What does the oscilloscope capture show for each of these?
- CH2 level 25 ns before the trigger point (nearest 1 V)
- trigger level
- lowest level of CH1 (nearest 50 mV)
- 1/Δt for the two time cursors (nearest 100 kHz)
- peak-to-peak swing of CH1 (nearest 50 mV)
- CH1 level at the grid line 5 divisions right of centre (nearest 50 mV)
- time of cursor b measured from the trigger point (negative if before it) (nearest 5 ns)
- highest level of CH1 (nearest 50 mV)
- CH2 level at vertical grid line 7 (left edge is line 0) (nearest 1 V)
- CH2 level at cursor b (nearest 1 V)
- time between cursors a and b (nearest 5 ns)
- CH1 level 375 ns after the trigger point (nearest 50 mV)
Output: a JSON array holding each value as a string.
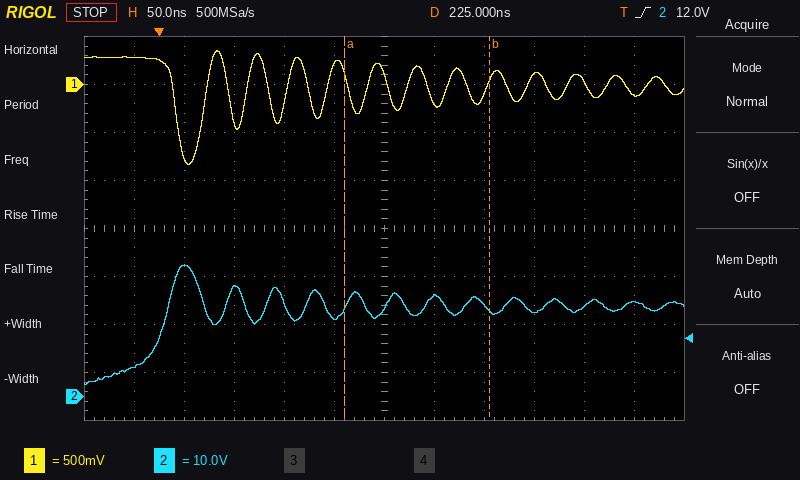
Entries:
["6 V", "12.0 V", "-850 mV", "6.9 MHz", "1.20 V", "-100 mV", "+330 ns", "350 mV", "21 V", "18 V", "145 ns", "100 mV"]
